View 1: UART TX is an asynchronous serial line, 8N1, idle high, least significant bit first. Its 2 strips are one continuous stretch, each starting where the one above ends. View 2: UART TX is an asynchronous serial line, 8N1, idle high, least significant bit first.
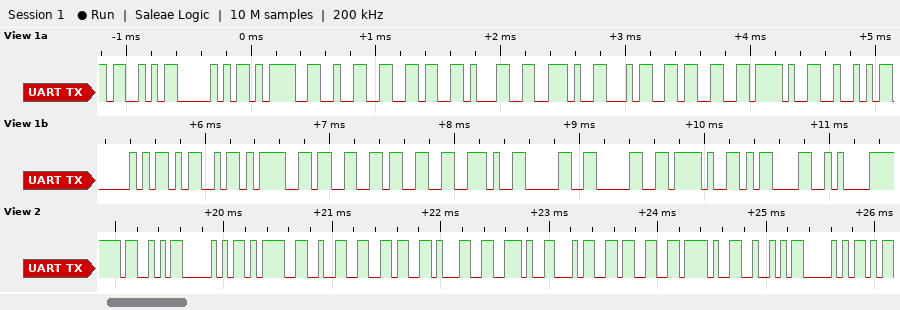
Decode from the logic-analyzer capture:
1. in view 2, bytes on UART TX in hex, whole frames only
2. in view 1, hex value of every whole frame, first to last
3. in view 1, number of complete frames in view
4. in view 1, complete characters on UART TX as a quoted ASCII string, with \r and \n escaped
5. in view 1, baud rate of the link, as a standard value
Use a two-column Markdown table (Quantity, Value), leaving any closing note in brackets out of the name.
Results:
| Quantity | Value |
|---|---|
| in view 2, bytes on UART TX in hex, whole frames only | 53 50 3D 32 36 31 2E 34 33 2F 52 50 |
| in view 1, hex value of every whole frame, first to last | 0x53 0x50 0x3D 0x32 0x36 0x31 0x2E 0x34 0x33 0x2F 0x52 0x50 0x4D 0x3D 0x33 0x33 0x2E 0x30 0x30 0x2F 0x0D 0x0A |
| in view 1, number of complete frames in view | 22 |
| in view 1, complete characters on UART TX as a quoted ASCII string, with \r and \n escaped | "SP=261.43/RPM=33.00/\r\n" |
| in view 1, baud rate of the link, as a standard value | 19200 baud |
